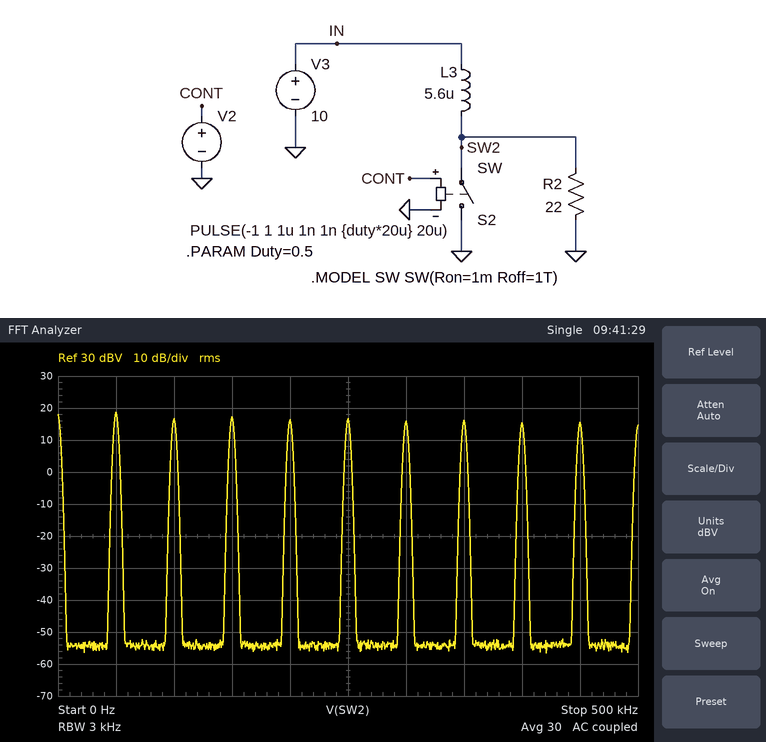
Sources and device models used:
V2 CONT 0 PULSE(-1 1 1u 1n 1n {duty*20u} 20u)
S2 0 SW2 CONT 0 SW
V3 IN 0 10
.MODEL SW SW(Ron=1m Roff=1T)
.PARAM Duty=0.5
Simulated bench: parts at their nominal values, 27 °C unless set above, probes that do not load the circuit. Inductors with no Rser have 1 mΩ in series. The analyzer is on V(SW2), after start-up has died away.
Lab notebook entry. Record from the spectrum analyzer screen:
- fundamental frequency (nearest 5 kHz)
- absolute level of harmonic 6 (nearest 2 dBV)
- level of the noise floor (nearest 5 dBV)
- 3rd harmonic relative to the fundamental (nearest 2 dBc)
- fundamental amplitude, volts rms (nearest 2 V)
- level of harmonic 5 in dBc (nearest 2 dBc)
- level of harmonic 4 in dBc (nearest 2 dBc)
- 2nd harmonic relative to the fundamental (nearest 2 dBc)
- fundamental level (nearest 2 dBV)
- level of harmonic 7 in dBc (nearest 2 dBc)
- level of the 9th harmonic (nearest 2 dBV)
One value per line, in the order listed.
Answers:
50 kHz
16 dBV
-55 dBV
-2 dBc
8 V
-2 dBc
-2 dBc
-2 dBc
18 dBV
-2 dBc
16 dBV
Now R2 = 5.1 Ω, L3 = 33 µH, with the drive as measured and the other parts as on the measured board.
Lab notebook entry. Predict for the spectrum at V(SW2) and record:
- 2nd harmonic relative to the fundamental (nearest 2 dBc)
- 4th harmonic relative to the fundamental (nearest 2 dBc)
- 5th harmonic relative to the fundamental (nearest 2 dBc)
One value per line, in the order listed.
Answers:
-14 dBc
-20 dBc
-14 dBc
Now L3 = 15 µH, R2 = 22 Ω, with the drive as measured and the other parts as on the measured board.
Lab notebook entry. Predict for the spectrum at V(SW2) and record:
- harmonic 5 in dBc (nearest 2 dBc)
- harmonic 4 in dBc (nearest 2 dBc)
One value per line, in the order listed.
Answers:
-4 dBc
-4 dBc
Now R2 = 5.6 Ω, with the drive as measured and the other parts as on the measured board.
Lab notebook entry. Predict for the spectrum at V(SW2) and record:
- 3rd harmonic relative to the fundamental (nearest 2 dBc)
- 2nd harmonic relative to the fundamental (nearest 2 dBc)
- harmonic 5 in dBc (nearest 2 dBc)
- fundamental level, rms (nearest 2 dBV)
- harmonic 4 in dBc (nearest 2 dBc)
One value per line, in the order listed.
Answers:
-4 dBc
-4 dBc
-6 dBc
20 dBV
-6 dBc
